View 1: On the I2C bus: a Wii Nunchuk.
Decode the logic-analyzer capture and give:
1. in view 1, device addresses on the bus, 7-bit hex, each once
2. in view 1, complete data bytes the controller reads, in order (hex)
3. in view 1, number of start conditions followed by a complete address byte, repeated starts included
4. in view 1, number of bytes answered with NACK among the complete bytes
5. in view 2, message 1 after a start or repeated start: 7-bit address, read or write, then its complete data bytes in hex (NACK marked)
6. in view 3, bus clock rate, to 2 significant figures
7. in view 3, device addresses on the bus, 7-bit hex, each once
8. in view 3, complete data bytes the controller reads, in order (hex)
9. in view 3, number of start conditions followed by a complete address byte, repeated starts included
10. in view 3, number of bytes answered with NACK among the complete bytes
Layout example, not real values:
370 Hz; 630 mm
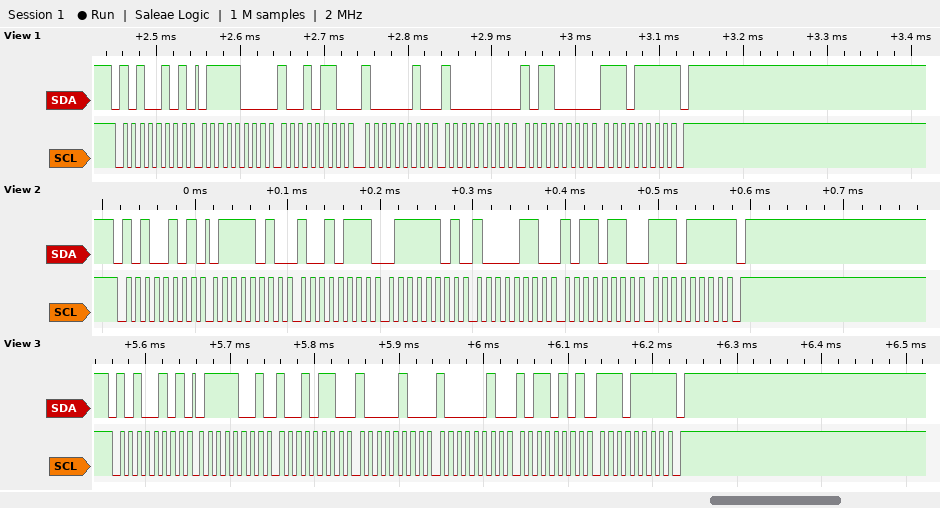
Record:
0x52; 78 96 82 80 B0 EF; 1; 1; 0x52 read: 7A 97 7D 86 B6 EF NACK; 100 kHz; 0x52; 79 96 84 82 B5 EF; 1; 1
